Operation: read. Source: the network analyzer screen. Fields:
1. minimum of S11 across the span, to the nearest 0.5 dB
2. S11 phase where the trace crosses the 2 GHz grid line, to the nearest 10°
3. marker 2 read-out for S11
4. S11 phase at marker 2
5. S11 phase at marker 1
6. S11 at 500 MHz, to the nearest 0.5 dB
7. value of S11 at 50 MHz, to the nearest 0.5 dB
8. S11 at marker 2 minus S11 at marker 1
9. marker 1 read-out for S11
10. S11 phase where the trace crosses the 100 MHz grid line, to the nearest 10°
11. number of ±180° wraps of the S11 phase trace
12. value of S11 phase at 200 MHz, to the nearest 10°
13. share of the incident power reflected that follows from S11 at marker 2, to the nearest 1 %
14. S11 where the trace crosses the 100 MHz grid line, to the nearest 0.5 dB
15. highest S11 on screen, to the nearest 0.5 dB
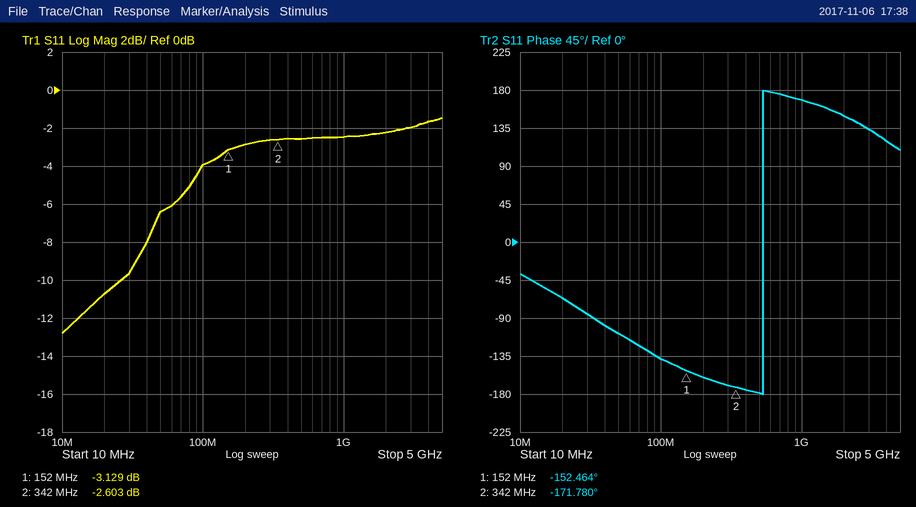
-13.0 dB
150°
-2.603 dB
-171.780°
-152.464°
-2.5 dB
-6.5 dB
0.526 dB
-3.129 dB
-140°
1
-160°
55 %
-4.0 dB
-1.5 dB
